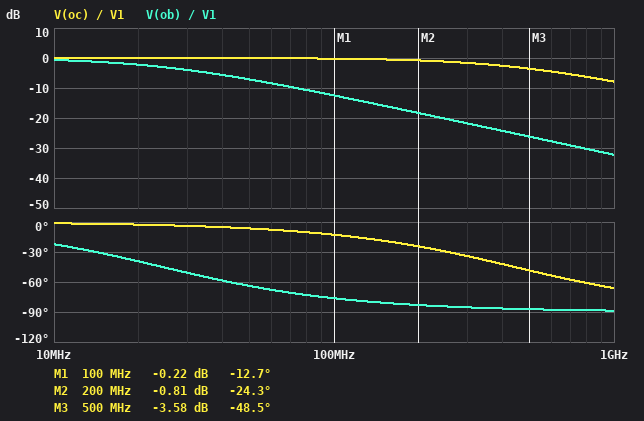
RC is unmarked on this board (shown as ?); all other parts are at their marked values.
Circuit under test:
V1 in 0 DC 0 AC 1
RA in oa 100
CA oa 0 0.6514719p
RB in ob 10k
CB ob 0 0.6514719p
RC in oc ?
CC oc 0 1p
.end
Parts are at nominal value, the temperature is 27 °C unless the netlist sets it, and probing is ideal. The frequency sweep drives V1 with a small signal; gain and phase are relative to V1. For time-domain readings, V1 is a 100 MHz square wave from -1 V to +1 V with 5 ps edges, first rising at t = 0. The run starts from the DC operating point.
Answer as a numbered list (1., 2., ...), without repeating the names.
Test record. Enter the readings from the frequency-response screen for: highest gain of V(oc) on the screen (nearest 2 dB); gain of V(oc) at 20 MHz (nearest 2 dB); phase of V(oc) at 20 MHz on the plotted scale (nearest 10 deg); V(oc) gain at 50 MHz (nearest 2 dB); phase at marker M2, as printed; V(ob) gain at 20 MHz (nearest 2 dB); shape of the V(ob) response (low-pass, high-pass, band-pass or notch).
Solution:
1. 0 dB
2. 0 dB
3. 0 deg
4. 0 dB
5. -24.3 deg
6. -2 dB
7. low-pass
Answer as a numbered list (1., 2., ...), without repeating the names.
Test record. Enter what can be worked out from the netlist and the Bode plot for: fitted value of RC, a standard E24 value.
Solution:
1. 360 Ω
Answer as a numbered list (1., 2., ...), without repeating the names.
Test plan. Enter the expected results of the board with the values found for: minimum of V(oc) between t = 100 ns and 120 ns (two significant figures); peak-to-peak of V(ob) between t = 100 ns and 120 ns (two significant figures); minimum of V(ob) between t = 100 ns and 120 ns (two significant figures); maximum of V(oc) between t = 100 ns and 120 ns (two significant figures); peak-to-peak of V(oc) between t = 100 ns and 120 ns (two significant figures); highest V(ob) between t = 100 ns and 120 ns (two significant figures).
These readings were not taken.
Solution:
1. -1.0 V
2. 730 mV
3. -370 mV
4. 1.0 V
5. 2.0 V
6. 370 mV
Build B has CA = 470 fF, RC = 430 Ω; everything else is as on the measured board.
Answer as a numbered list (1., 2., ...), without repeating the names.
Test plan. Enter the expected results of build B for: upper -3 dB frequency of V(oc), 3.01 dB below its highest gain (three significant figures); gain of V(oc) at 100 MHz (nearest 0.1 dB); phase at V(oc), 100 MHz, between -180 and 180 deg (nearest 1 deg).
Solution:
1. 370 MHz
2. -0.3 dB
3. -15 deg
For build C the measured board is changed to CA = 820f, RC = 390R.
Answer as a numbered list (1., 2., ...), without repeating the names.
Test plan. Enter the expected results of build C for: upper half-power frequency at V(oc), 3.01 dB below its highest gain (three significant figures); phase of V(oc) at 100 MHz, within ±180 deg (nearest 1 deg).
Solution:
1. 408 MHz
2. -14 deg
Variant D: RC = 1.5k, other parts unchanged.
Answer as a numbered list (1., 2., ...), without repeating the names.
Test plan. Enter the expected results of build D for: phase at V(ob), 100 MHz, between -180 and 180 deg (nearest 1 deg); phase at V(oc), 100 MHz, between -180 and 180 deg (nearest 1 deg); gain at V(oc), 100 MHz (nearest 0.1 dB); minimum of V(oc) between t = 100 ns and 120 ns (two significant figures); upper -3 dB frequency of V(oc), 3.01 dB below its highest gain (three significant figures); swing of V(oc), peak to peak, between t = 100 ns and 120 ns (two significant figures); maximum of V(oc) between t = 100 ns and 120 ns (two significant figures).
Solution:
1. -76 deg
2. -43 deg
3. -2.8 dB
4. -930 mV
5. 106 MHz
6. 1.9 V
7. 930 mV
